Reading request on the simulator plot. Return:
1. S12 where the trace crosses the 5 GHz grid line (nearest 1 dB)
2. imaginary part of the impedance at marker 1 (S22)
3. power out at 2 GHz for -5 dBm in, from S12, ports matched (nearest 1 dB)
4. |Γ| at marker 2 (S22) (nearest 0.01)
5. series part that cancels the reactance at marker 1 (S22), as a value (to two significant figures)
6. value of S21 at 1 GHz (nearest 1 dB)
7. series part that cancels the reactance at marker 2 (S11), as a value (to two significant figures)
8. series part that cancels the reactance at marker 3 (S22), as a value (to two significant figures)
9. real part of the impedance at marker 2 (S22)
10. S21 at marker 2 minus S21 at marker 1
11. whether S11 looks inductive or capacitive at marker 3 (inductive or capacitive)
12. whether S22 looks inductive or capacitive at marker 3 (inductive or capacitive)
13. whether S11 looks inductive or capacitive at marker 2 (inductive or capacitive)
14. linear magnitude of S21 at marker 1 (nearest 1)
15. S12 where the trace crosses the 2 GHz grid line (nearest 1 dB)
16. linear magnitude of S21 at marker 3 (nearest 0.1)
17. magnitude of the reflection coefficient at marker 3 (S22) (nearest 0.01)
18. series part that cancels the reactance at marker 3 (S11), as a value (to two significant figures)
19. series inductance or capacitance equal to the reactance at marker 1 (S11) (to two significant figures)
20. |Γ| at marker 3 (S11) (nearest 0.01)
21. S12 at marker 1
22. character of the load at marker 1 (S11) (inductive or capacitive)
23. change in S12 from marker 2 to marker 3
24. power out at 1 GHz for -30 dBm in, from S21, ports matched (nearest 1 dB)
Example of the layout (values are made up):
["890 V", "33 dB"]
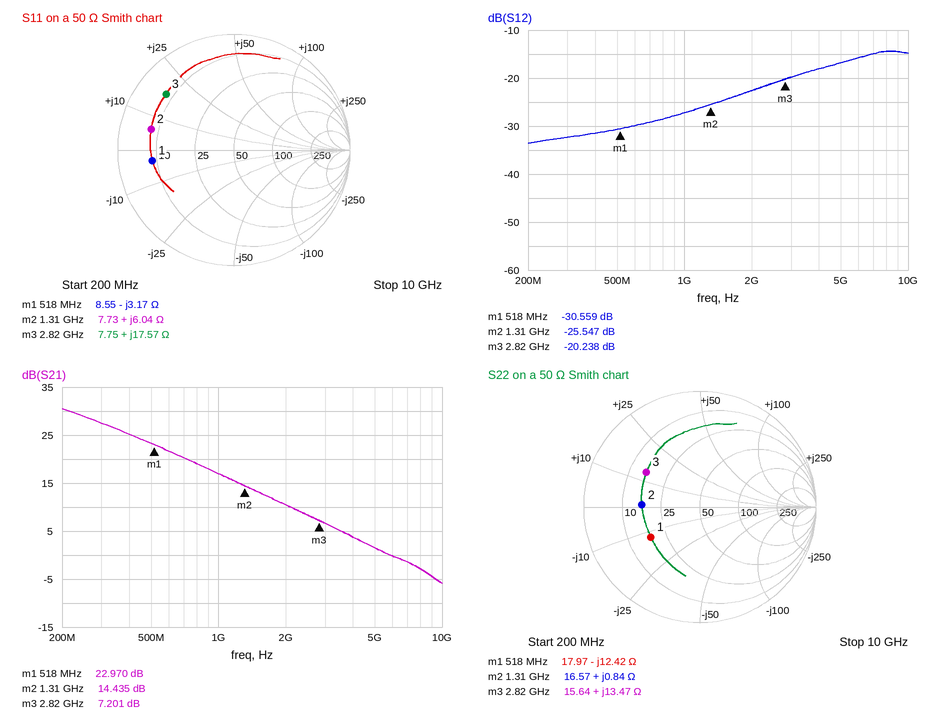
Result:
["-17 dB", "-12.42 Ω", "-28 dBm", "0.50", "3.8 nH", "17 dB", "20 pF", "4.2 pF", "16.57 Ω", "-8.535 dB", "inductive", "inductive", "inductive", "14", "-23 dB", "2.3", "0.55", "3.2 pF", "97 pF", "0.76", "-30.559 dB", "capacitive", "5.309 dB", "-13 dBm"]
